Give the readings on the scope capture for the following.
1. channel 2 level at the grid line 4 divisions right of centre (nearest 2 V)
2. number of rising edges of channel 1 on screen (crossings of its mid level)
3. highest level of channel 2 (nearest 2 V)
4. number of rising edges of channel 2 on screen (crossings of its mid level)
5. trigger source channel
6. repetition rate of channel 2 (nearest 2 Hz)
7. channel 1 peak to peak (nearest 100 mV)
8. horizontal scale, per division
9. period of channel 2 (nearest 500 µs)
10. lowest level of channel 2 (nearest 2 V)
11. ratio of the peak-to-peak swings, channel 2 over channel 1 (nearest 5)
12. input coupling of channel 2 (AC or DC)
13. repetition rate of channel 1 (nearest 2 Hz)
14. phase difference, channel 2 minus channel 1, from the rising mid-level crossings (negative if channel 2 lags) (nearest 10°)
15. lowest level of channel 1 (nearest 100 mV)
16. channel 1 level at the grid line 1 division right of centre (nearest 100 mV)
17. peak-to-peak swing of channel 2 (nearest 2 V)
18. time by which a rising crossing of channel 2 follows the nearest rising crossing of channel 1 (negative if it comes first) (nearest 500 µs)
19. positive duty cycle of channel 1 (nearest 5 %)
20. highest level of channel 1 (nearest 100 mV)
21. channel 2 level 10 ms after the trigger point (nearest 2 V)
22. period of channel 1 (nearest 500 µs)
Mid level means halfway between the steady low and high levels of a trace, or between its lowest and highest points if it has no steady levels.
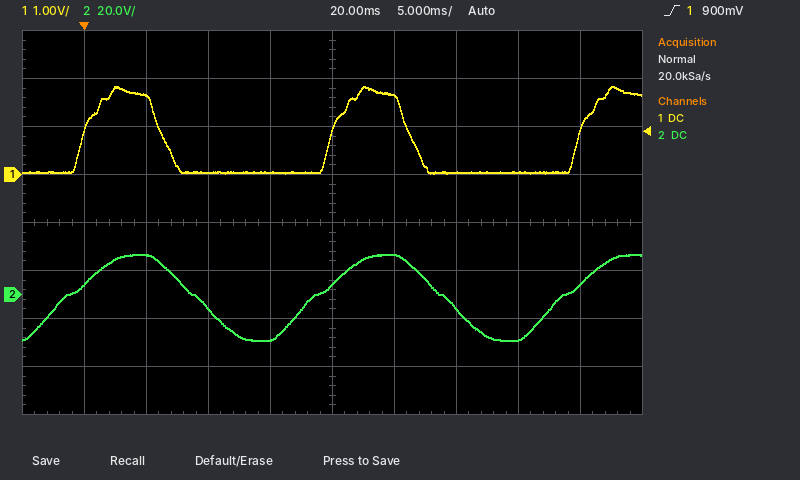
4 V
3
16 V
3
channel 1
50 Hz
1.8 V
5 ms
20.0 ms
-20 V
20
DC
50 Hz
+30°
0.0 V
1.6 V
36 V
-1.5 ms
30 %
1.8 V
-6 V
20.0 ms
